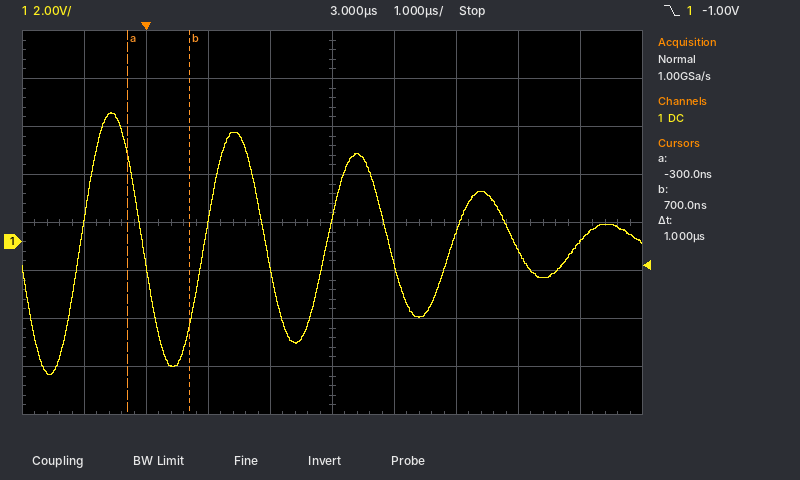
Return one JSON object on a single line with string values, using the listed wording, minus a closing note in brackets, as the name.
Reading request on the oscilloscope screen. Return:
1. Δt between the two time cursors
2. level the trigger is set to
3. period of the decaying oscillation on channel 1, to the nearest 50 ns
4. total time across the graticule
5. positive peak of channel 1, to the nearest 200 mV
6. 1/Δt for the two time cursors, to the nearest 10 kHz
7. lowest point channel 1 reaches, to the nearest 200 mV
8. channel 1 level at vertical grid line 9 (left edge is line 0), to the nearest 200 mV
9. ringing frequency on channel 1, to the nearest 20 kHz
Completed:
{"Δt between the two time cursors": "1 µs", "level the trigger is set to": "-1.00 V", "period of the decaying oscillation on channel 1, to the nearest 50 ns": "2.00 µs", "total time across the graticule": "10 µs", "positive peak of channel 1, to the nearest 200 mV": "5.4 V", "1/Δt for the two time cursors, to the nearest 10 kHz": "1.00 MHz", "lowest point channel 1 reaches, to the nearest 200 mV": "-5.6 V", "channel 1 level at vertical grid line 9 (left edge is line 0), to the nearest 200 mV": "0.0 V", "ringing frequency on channel 1, to the nearest 20 kHz": "500 kHz"}
